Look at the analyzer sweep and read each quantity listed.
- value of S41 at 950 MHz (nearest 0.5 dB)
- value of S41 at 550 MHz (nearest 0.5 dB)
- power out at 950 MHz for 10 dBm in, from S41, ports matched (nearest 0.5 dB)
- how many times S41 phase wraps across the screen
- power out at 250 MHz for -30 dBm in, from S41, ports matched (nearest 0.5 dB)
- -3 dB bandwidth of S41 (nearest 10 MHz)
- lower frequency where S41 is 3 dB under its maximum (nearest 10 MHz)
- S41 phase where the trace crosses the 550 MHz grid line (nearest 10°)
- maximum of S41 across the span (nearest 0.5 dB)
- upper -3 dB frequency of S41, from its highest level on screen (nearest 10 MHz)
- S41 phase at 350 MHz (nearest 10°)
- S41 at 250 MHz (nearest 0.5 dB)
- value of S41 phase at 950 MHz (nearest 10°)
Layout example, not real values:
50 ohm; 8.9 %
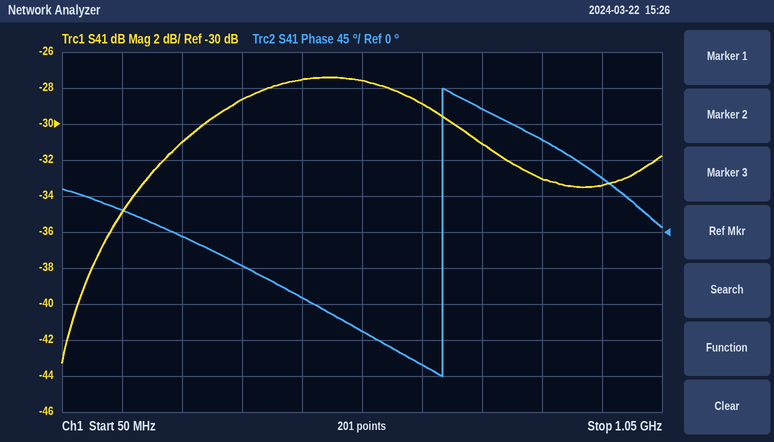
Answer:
-33.5 dB; -27.5 dB; -23.5 dBm; 1; -61.0 dBm; 450 MHz; 270 MHz; -120°; -27.5 dB; 720 MHz; -40°; -31.0 dB; 70°
